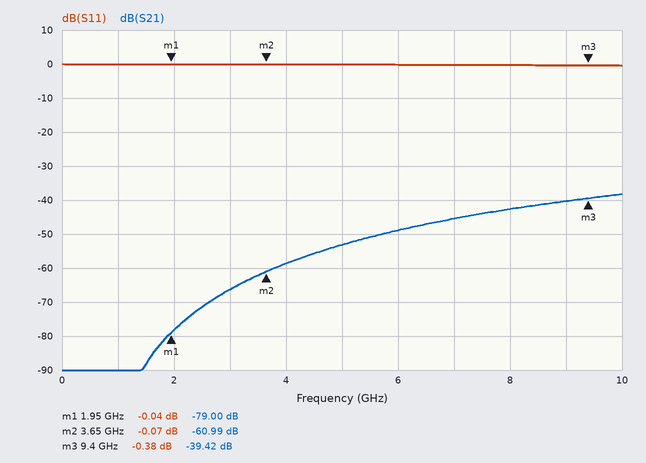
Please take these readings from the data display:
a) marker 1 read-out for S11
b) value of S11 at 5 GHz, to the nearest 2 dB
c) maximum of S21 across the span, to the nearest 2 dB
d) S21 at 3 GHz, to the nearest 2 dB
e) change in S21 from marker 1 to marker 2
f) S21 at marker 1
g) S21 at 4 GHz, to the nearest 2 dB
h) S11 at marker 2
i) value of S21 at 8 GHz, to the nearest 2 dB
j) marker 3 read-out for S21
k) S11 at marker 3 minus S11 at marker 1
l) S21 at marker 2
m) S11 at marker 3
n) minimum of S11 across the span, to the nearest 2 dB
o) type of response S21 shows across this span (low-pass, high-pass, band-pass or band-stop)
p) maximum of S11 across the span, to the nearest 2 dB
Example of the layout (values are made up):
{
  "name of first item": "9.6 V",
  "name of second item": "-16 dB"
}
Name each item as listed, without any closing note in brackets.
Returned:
{
  "marker 1 read-out for S11": "-0.04 dB",
  "value of S11 at 5 GHz, to the nearest 2 dB": "0 dB",
  "maximum of S21 across the span, to the nearest 2 dB": "-38 dB",
  "S21 at 3 GHz, to the nearest 2 dB": "-66 dB",
  "change in S21 from marker 1 to marker 2": "18.01 dB",
  "S21 at marker 1": "-79.00 dB",
  "S21 at 4 GHz, to the nearest 2 dB": "-58 dB",
  "S11 at marker 2": "-0.07 dB",
  "value of S21 at 8 GHz, to the nearest 2 dB": "-42 dB",
  "marker 3 read-out for S21": "-39.42 dB",
  "S11 at marker 3 minus S11 at marker 1": "-0.34 dB",
  "S21 at marker 2": "-60.99 dB",
  "S11 at marker 3": "-0.38 dB",
  "minimum of S11 across the span, to the nearest 2 dB": "0 dB",
  "type of response S21 shows across this span": "high-pass",
  "maximum of S11 across the span, to the nearest 2 dB": "0 dB"
}
